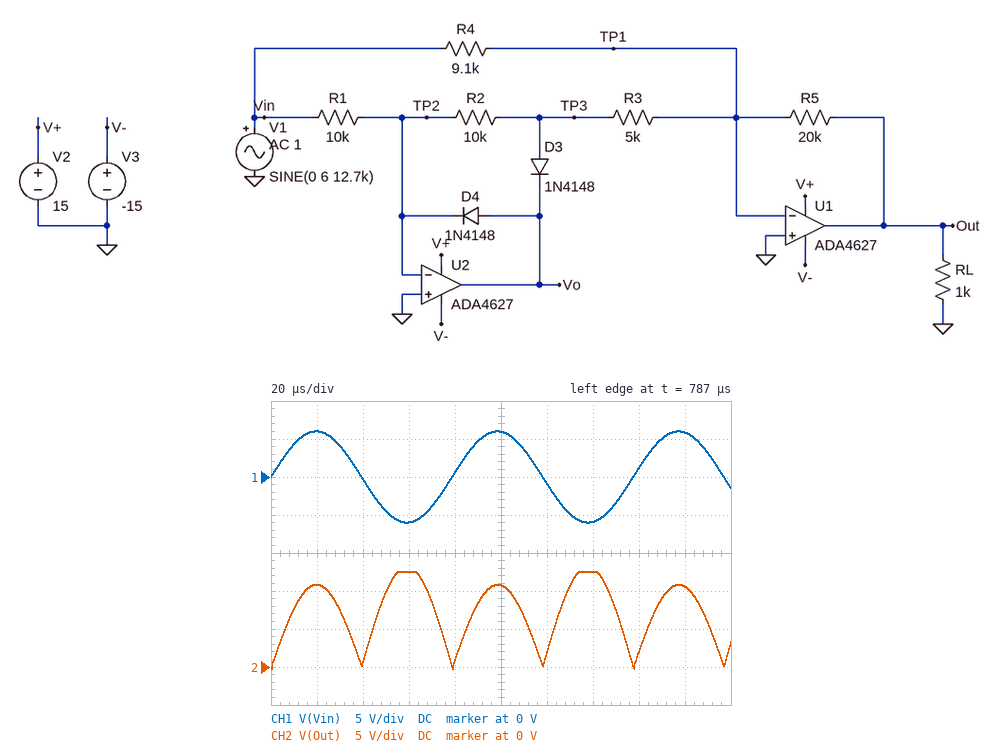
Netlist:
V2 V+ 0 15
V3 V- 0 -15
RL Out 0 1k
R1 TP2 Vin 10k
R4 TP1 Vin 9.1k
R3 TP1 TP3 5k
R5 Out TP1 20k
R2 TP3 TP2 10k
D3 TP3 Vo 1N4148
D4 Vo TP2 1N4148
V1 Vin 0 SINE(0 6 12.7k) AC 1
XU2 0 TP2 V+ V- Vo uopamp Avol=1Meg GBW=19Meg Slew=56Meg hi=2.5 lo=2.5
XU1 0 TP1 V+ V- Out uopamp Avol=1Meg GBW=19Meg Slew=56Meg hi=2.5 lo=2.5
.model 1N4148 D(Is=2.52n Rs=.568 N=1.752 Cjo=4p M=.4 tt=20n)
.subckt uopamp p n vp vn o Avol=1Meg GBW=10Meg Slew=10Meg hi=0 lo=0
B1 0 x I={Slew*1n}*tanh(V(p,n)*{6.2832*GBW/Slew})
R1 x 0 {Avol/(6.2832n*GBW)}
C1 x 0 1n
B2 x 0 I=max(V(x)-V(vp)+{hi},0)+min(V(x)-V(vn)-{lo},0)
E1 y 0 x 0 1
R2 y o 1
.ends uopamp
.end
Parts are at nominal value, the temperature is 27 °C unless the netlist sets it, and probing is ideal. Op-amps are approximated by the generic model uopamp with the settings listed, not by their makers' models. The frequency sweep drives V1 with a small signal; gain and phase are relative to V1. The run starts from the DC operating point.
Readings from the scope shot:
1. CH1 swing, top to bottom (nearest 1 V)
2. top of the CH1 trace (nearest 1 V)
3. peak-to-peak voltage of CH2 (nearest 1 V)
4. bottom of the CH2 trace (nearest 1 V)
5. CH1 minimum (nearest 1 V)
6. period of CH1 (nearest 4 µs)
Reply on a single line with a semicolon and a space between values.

12 V; 6 V; 13 V; 0 V; -6 V; 80 µs
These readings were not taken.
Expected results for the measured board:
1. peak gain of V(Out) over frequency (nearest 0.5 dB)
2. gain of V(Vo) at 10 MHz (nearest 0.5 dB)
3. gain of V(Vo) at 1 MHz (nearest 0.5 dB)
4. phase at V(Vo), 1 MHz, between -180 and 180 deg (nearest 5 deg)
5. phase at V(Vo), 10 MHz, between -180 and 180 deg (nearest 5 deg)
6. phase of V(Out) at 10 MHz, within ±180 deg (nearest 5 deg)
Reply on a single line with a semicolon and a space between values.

4.0 dB; -11.0 dB; 7.5 dB; 90 deg; 75 deg; 110 deg
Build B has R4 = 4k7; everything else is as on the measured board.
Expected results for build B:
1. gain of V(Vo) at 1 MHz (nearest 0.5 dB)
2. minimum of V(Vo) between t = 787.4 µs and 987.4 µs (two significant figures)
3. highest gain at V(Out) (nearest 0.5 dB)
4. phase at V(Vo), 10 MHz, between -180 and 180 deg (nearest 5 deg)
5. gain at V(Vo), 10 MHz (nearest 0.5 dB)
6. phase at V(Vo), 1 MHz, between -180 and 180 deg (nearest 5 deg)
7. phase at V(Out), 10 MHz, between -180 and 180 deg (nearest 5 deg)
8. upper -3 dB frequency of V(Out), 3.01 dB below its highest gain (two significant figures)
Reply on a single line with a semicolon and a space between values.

8.0 dB; -6.6 V; 11.0 dB; 70 deg; -10.5 dB; 95 deg; 100 deg; 2.9 MHz
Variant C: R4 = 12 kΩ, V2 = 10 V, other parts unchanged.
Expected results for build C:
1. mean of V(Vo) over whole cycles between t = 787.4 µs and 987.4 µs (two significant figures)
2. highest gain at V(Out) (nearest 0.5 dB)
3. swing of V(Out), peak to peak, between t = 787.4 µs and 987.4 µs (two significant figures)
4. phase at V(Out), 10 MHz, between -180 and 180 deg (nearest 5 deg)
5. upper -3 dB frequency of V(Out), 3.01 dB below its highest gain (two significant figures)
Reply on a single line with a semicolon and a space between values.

-1.9 V; 0.5 dB; 7.7 V; 115 deg; 6.1 MHz
